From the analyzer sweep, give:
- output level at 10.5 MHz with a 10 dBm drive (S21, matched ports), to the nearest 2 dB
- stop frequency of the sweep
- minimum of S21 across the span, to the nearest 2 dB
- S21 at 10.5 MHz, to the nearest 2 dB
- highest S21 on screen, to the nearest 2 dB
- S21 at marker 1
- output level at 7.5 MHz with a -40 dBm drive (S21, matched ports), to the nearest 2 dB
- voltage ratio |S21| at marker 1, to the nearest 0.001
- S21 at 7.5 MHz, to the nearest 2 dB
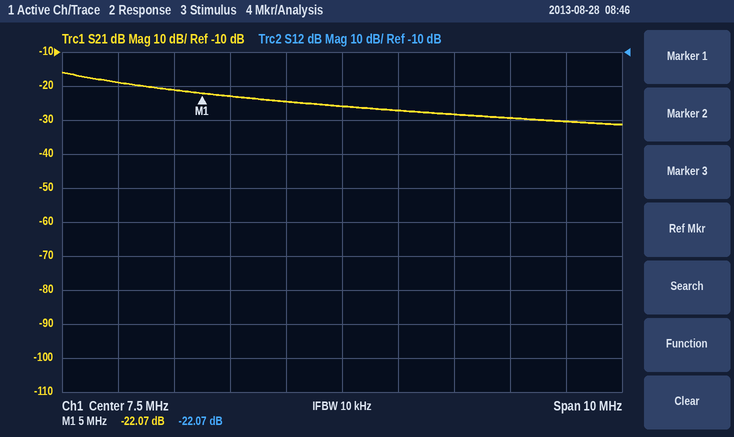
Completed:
-20 dBm
12.5 MHz
-32 dB
-30 dB
-16 dB
-22.07 dB
-66 dBm
0.079
-26 dB
